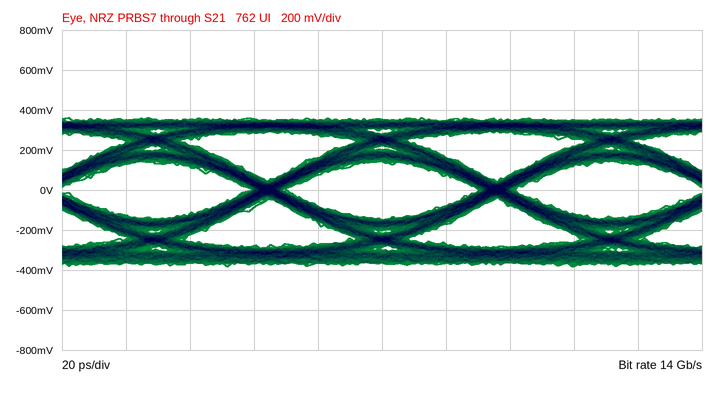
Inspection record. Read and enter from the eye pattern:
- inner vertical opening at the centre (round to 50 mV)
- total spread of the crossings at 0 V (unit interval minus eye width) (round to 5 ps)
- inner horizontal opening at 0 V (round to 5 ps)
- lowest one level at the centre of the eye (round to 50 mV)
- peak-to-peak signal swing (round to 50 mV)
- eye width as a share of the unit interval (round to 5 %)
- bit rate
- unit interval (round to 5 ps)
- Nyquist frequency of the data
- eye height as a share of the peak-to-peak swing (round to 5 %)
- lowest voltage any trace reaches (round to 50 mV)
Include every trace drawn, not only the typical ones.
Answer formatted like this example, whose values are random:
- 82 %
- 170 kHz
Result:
- 300 mV
- 10 ps
- 60 ps
- 150 mV
- 750 mV
- 85 %
- 14 Gb/s
- 70 ps
- 7 GHz
- 40 %
- -400 mV
